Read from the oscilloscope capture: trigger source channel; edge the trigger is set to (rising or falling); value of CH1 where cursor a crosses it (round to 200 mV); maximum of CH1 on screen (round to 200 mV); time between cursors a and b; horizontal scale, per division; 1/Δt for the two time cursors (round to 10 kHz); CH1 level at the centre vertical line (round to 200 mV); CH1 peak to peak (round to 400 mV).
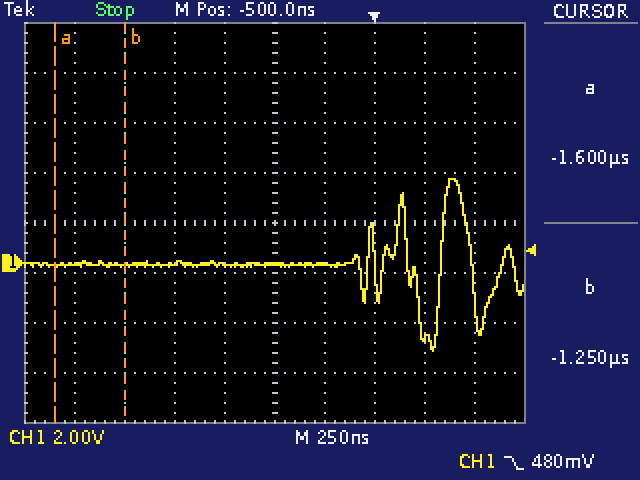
CH1
falling
0.0 V
3.4 V
350 ns
250 ns
2.86 MHz
0.0 V
6.8 V
